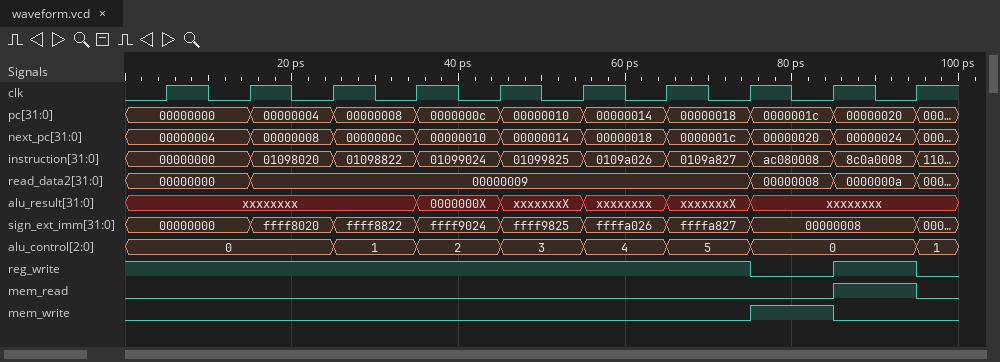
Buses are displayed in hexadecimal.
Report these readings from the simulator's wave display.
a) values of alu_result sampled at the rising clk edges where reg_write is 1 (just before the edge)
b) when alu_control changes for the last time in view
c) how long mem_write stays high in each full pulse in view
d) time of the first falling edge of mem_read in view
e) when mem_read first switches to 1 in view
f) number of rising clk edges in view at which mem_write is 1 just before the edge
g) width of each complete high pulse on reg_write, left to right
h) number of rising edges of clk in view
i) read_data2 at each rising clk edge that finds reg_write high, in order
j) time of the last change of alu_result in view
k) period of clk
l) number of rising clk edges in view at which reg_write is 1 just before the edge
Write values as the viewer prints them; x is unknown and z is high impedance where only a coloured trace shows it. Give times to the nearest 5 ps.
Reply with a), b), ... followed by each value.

a) xxxxxxxx, xxxxxxxx, xxxxxxxx, xxxxxxxx, 0000000X, xxxxxxxX, xxxxxxxx, xxxxxxxX, xxxxxxxx
b) 95 ps
c) 10 ps
d) 95 ps
e) 85 ps
f) 1
g) 10 ps
h) 10
i) 00000000, 00000000, 00000009, 00000009, 00000009, 00000009, 00000009, 00000009, 0000000a
j) 75 ps
k) 10 ps
l) 9
